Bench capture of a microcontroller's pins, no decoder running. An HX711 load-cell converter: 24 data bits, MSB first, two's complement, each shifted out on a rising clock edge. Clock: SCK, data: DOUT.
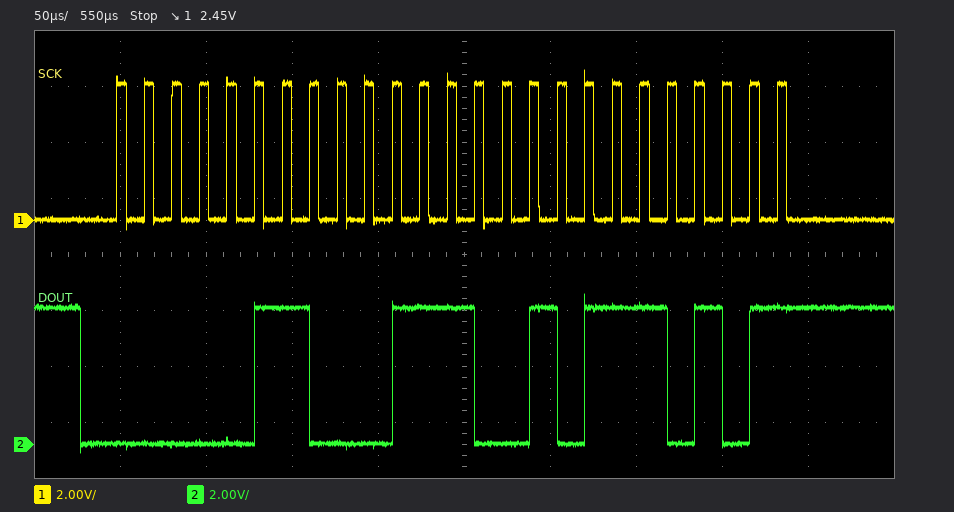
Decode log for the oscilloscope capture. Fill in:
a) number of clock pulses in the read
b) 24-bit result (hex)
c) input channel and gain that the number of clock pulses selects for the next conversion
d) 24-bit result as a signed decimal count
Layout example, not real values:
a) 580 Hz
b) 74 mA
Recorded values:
a) 25
b) 0x063975
c) channel A, gain 128
d) 407925
